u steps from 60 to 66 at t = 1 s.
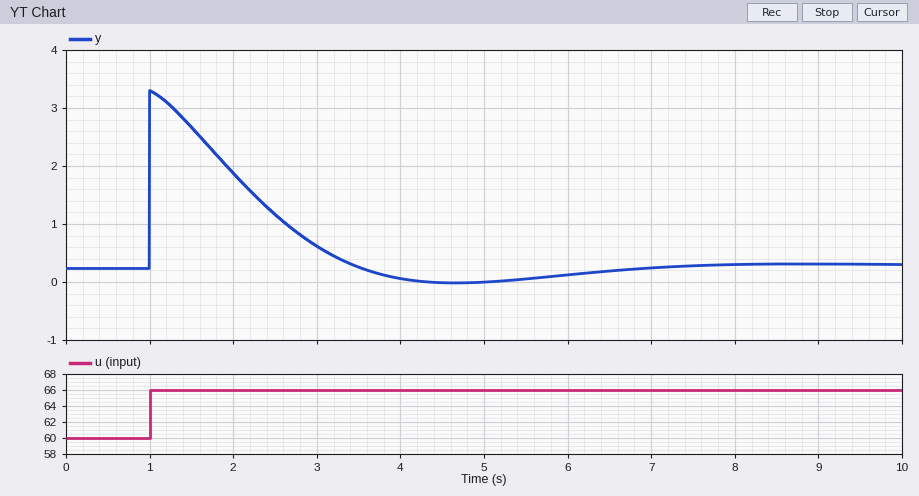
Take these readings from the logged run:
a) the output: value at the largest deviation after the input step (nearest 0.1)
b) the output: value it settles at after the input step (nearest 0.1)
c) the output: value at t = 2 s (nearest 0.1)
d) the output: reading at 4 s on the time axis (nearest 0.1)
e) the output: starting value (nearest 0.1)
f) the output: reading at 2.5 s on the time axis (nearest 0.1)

3.3
0.3
1.9
0.1
0.2
1.2
